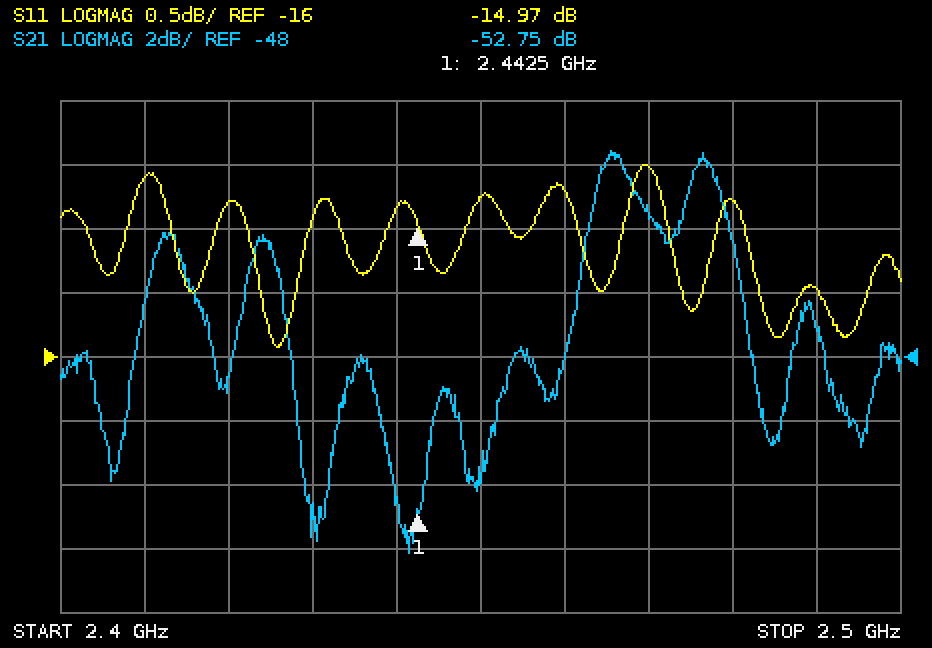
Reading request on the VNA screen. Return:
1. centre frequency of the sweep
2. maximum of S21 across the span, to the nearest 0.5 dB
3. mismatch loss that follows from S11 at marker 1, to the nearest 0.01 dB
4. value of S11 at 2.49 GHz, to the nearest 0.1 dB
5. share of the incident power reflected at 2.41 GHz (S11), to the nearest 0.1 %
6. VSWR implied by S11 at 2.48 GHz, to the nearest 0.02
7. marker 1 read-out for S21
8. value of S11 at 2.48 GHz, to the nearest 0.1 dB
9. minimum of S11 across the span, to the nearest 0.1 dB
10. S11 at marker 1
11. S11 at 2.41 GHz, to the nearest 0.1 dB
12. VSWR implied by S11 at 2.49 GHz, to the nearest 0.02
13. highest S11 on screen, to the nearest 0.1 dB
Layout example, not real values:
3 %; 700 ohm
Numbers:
2.45 GHz; -41.5 dB; 0.14 dB; -15.5 dB; 3.5 %; 1.44; -52.75 dB; -14.8 dB; -15.9 dB; -14.97 dB; -14.6 dB; 1.40; -14.5 dB
